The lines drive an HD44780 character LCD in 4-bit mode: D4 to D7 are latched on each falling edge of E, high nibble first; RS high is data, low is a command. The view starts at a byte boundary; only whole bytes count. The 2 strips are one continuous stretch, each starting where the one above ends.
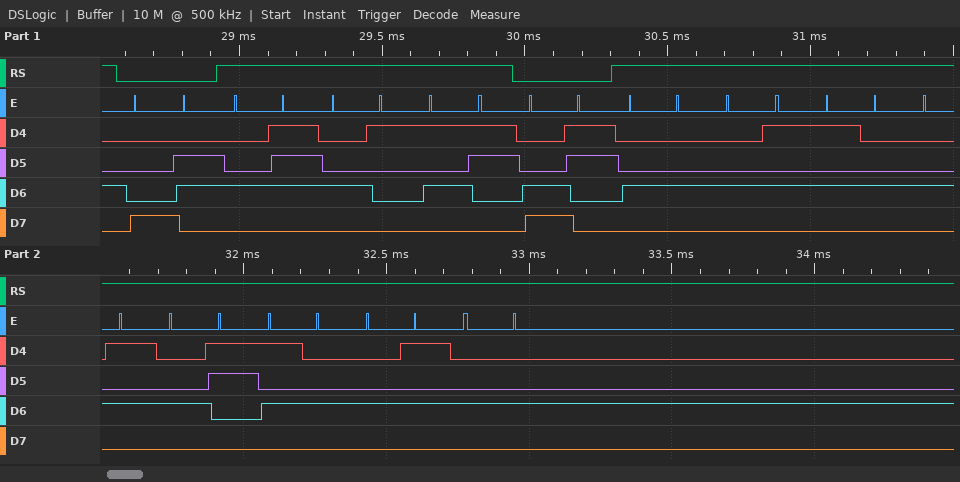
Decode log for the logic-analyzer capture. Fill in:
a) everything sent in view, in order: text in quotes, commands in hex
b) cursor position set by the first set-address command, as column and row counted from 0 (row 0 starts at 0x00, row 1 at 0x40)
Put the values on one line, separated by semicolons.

0x86 "GAS" 0xC3 "DETECTED"; column 6, row 0
